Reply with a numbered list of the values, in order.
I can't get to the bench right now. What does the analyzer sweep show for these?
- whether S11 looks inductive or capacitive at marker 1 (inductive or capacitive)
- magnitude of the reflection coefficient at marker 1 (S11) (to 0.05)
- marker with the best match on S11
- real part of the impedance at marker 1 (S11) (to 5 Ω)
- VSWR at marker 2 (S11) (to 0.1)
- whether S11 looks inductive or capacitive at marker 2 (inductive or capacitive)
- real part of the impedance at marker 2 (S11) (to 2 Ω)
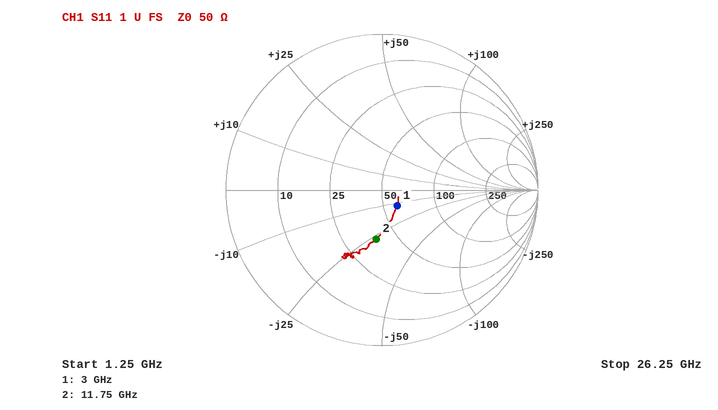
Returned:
1. capacitive
2. 0.15
3. marker 1
4. 60 Ω
5. 1.9
6. capacitive
7. 38 Ω
